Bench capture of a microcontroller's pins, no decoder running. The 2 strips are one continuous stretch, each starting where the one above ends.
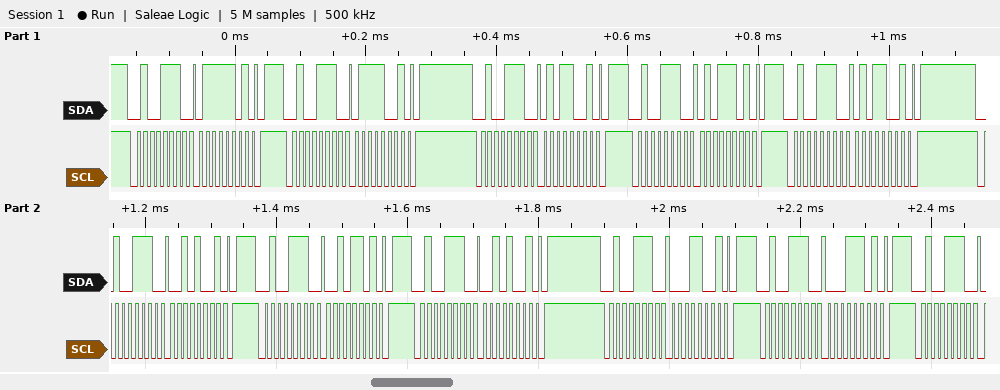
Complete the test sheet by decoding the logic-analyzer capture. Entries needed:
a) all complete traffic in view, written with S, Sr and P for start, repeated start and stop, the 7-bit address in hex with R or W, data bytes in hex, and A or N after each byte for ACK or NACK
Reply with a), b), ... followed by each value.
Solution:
a) S 27W A 7D A P S 27W A 79 A P S 27W A 59 A P S 27W A 5D A P S 27W A 59 A P S 27W A 29 A P S 27W A 2D A P S 27W A 29 A P S 27W A 19 A P S 27W A 1D A P S 27W A
